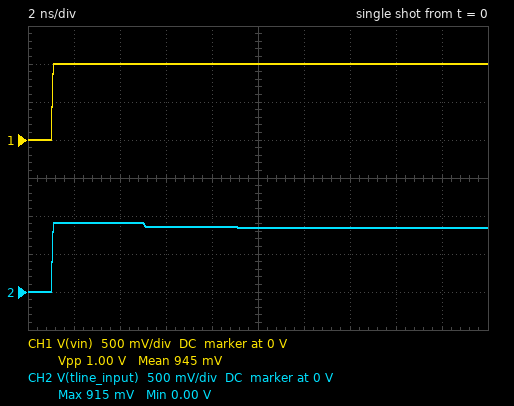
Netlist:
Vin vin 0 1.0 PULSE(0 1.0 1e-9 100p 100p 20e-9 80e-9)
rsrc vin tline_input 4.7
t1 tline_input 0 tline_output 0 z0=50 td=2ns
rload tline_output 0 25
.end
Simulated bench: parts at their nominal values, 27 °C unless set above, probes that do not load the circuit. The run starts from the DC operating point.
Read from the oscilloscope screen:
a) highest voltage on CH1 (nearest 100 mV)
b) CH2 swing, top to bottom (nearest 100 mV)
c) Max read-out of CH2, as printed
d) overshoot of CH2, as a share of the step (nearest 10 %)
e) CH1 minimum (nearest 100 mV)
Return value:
1.0 V
900 mV
915 mV
10 %
0 V
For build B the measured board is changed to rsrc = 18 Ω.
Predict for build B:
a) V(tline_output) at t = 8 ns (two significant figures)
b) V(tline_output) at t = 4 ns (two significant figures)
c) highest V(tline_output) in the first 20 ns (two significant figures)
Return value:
570 mV
490 mV
580 mV
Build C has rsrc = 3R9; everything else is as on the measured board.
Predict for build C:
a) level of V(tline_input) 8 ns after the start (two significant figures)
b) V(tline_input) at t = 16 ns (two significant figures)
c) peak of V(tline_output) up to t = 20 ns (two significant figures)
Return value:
880 mV
870 mV
860 mV
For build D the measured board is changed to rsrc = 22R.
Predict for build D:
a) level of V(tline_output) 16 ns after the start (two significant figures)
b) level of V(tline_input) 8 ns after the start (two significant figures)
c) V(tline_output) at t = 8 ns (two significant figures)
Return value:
530 mV
550 mV
520 mV
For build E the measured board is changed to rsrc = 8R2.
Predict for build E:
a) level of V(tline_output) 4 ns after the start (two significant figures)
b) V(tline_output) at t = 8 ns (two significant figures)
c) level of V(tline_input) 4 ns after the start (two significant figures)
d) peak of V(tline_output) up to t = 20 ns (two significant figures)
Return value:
570 mV
710 mV
860 mV
750 mV
